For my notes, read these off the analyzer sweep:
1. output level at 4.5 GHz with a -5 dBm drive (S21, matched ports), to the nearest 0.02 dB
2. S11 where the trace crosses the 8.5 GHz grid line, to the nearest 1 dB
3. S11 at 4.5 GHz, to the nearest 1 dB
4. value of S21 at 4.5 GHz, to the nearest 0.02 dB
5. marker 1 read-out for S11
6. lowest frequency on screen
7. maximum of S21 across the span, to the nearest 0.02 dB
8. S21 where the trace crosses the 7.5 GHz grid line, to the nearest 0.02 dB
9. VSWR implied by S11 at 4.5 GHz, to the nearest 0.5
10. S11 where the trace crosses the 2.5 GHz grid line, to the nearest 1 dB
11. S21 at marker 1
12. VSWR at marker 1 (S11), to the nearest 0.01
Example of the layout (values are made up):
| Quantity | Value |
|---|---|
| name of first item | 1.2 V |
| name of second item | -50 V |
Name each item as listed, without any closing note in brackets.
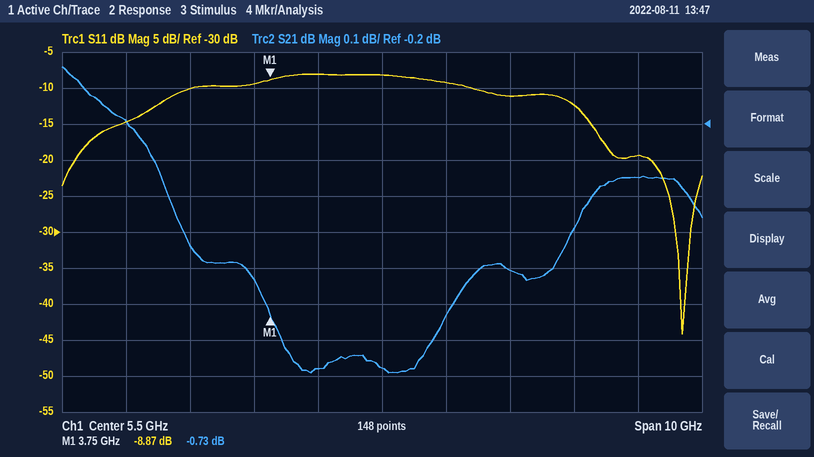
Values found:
| Quantity | Value |
|---|---|
| output level at 4.5 GHz with a -5 dBm drive (S21, matched ports), to the nearest 0.02 dB | -5.88 dBm |
| S11 where the trace crosses the 8.5 GHz grid line, to the nearest 1 dB | -12 dB |
| S11 at 4.5 GHz, to the nearest 1 dB | -8 dB |
| value of S21 at 4.5 GHz, to the nearest 0.02 dB | -0.88 dB |
| marker 1 read-out for S11 | -8.87 dB |
| lowest frequency on screen | 500 MHz |
| maximum of S21 across the span, to the nearest 0.02 dB | -0.04 dB |
| S21 where the trace crosses the 7.5 GHz grid line, to the nearest 0.02 dB | -0.60 dB |
| VSWR implied by S11 at 4.5 GHz, to the nearest 0.5 | 2.5 |
| S11 where the trace crosses the 2.5 GHz grid line, to the nearest 1 dB | -10 dB |
| S21 at marker 1 | -0.73 dB |
| VSWR at marker 1 (S11), to the nearest 0.01 | 2.13 |
